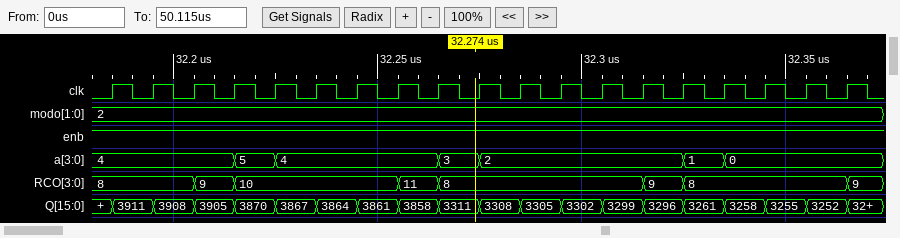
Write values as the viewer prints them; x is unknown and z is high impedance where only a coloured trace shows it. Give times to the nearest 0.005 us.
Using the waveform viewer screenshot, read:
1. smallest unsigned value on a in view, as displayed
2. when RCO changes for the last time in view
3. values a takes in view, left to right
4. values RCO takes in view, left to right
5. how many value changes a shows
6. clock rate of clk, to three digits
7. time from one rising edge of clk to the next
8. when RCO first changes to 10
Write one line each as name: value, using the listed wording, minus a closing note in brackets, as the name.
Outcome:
smallest unsigned value on a in view, as displayed: 0
when RCO changes for the last time in view: 32.365 us
values a takes in view, left to right: 4, 5, 4, 3, 2, 1, 0
values RCO takes in view, left to right: 8, 9, 10, 11, 8, 9, 8, 9
how many value changes a shows: 6
clock rate of clk, to three digits: 100 MHz
time from one rising edge of clk to the next: 0.01 us
when RCO first changes to 10: 32.215 us
